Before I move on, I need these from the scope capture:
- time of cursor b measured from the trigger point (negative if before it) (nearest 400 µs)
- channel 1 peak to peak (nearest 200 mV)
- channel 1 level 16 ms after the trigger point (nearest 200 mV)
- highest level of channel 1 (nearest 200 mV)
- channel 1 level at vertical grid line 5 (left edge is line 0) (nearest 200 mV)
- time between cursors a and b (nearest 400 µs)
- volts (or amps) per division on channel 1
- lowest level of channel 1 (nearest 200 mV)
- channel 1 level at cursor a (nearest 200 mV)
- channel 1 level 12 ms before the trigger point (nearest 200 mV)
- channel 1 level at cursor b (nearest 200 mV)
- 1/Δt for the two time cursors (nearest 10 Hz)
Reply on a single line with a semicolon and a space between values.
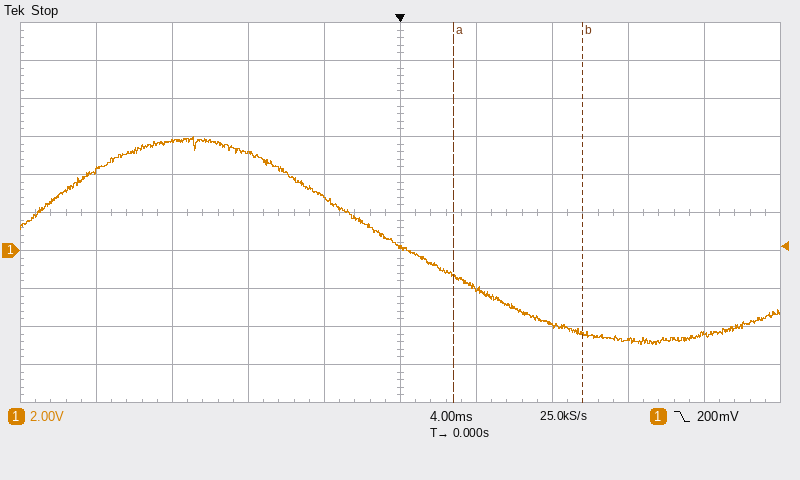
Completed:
+9.6 ms; 11.0 V; -4.4 V; 6.0 V; 200 mV; 6.8 ms; 2 V; -5.0 V; -1.4 V; 5.8 V; -4.4 V; 150 Hz
